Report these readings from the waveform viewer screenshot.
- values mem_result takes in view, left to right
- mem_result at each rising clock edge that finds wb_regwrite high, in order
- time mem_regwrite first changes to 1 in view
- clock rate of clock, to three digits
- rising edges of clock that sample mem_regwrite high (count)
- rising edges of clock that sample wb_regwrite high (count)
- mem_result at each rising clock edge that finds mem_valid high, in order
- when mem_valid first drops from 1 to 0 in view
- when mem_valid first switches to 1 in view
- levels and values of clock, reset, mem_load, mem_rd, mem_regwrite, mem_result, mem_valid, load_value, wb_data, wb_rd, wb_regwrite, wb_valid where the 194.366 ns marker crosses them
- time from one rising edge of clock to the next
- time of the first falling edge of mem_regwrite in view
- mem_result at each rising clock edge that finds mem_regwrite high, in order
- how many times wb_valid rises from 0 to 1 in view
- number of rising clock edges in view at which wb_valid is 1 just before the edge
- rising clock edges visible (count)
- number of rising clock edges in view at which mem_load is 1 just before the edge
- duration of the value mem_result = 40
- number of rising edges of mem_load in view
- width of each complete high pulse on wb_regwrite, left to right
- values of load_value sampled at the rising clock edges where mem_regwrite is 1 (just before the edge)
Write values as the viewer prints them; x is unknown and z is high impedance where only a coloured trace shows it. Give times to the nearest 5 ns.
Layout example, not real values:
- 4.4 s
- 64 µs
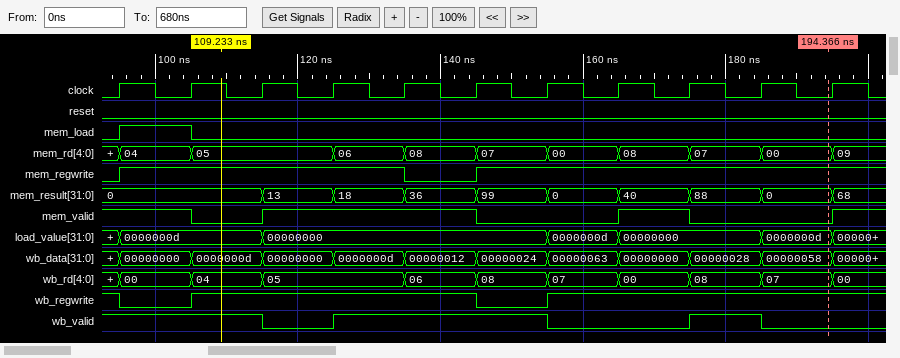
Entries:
- 0, 13, 18, 36, 99, 0, 40, 88, 0, 68
- 0, 0, 13, 18, 36, 0, 40, 88, 0
- 95 ns
- 100 MHz
- 9
- 9
- 0, 0, 13, 18, 36, 40
- 105 ns
- 115 ns
- clock=0, reset=0, mem_load=0, mem_rd=00, mem_regwrite=1, mem_result=0, mem_valid=0, load_value=0000000d, wb_data=00000058, wb_rd=07, wb_regwrite=1, wb_valid=0
- 10 ns
- 135 ns
- 0, 0, 13, 18, 99, 0, 40, 88, 0
- 2
- 7
- 11
- 1
- 10 ns
- 1
- 40 ns
- 0000000d, 0000000d, 00000000, 00000000, 00000000, 0000000d, 00000000, 00000000, 0000000d
